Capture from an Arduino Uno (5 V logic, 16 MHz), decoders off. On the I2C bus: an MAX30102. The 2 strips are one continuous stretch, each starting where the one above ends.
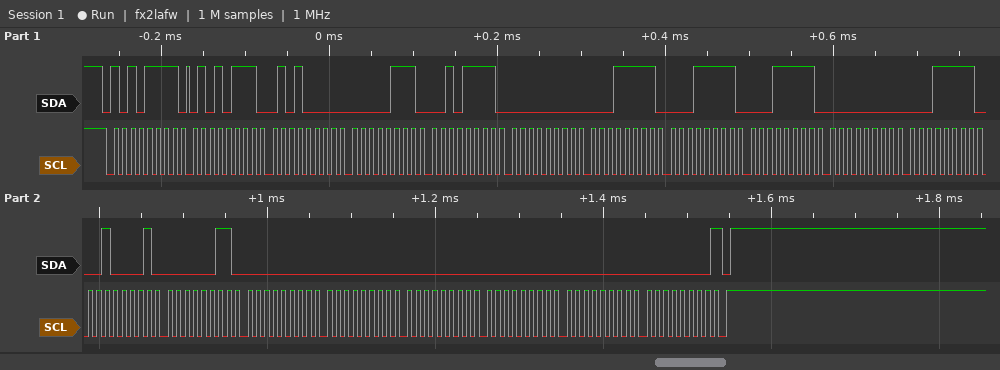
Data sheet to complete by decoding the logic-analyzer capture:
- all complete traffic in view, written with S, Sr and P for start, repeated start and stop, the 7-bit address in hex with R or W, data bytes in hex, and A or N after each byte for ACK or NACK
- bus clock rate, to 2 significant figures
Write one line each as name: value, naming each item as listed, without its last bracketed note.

all complete traffic in view, written with S, Sr and P for start, repeated start and stop, the 7-bit address in hex with R or W, data bytes in hex, and A or N after each byte for ACK or NACK: S 57R A 57 A 50 A 07 A 2F A 00 A 1F A 1F A 1F A 00 A 1F A 21 A 03 A 00 A 00 A 00 A 00 A 00 A 00 N P
bus clock rate, to 2 significant figures: 100 kHz
